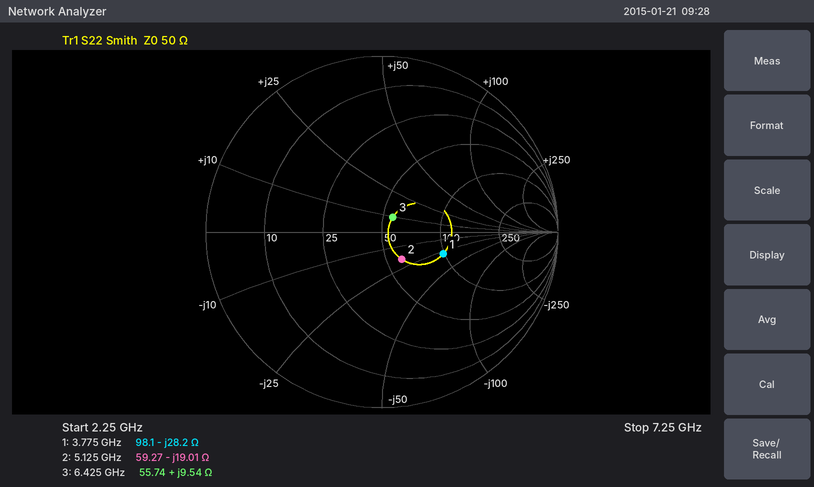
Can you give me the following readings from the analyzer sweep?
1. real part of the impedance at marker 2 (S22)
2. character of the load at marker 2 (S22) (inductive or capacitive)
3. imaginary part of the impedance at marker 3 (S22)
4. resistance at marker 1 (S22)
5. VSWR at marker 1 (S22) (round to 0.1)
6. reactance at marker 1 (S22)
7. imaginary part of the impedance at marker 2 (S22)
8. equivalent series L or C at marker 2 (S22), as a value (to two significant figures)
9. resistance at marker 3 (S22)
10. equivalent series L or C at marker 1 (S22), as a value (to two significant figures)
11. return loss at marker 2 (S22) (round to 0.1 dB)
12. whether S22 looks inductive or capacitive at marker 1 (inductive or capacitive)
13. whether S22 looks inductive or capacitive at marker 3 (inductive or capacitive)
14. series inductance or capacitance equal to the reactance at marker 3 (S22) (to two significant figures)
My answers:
59.27 Ω
capacitive
+9.54 Ω
98.1 Ω
2.2
-28.2 Ω
-19.01 Ω
1.6 pF
55.74 Ω
1.5 pF
14.4 dB
capacitive
inductive
240 pH
